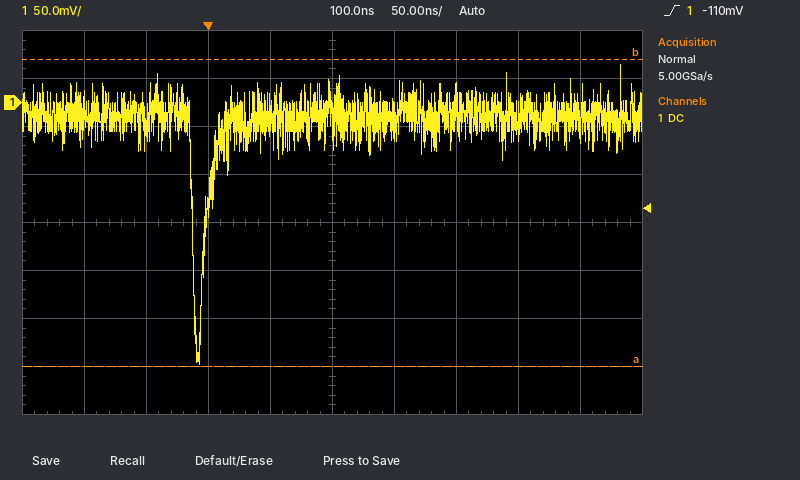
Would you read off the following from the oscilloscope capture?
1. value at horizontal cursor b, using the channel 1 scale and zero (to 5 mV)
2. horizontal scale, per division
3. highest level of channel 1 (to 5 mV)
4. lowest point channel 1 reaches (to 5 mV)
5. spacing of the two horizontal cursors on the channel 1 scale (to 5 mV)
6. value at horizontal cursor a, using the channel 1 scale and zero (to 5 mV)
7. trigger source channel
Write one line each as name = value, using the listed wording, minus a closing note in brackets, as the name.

value at horizontal cursor b, using the channel 1 scale and zero = 45 mV
horizontal scale, per division = 50 ns
highest level of channel 1 = 40 mV
lowest point channel 1 reaches = -275 mV
spacing of the two horizontal cursors on the channel 1 scale = 320 mV
value at horizontal cursor a, using the channel 1 scale and zero = -275 mV
trigger source channel = channel 1
